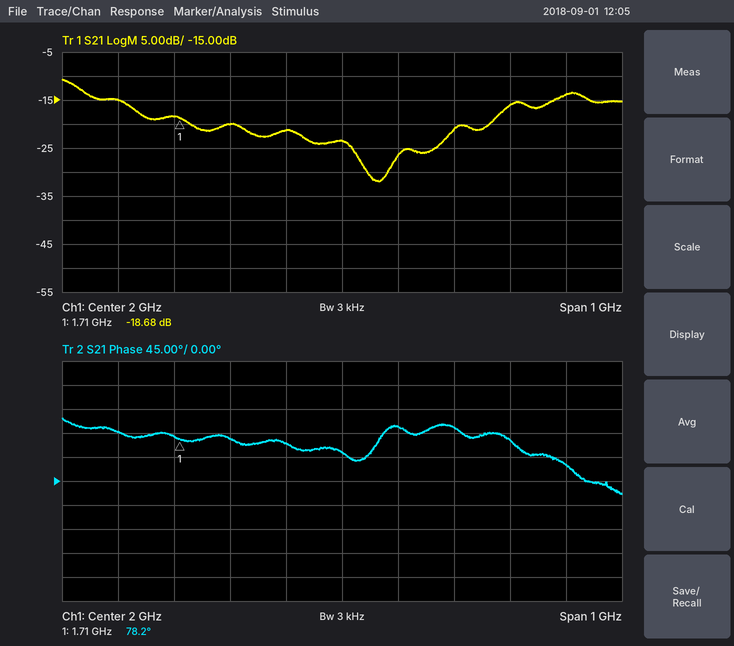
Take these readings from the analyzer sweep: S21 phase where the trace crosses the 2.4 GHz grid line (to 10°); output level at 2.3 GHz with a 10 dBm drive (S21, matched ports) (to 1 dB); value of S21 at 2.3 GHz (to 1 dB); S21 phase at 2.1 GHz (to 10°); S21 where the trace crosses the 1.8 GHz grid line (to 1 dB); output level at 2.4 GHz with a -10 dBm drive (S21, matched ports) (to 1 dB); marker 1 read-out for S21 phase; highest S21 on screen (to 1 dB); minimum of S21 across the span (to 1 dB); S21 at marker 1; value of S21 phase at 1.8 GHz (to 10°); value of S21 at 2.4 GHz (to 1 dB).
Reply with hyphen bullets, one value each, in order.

- 30°
- -6 dBm
- -16 dB
- 100°
- -20 dB
- -24 dBm
- 78.2°
- -11 dB
- -32 dB
- -18.68 dB
- 80°
- -14 dB
